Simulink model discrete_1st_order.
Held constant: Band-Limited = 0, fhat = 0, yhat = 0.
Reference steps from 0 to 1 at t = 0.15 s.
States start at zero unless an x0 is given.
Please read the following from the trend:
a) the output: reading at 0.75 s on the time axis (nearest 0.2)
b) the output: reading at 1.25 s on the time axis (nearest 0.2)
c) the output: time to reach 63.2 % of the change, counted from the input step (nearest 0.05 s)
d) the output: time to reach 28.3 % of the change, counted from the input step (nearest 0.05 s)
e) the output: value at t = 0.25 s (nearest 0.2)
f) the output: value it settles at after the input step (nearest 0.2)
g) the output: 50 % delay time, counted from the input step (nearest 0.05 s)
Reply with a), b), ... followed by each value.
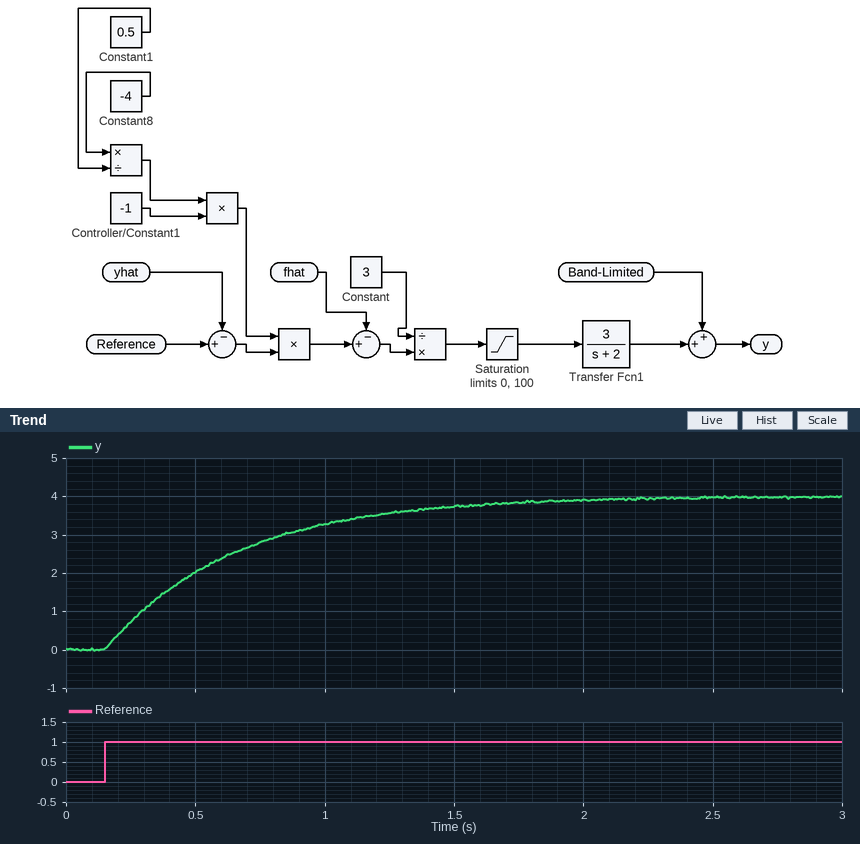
a) 2.8
b) 3.6
c) 0.50 s
d) 0.15 s
e) 0.8
f) 4.0
g) 0.35 s
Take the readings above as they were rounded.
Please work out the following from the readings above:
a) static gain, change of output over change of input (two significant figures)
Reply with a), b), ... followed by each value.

a) 4.0
